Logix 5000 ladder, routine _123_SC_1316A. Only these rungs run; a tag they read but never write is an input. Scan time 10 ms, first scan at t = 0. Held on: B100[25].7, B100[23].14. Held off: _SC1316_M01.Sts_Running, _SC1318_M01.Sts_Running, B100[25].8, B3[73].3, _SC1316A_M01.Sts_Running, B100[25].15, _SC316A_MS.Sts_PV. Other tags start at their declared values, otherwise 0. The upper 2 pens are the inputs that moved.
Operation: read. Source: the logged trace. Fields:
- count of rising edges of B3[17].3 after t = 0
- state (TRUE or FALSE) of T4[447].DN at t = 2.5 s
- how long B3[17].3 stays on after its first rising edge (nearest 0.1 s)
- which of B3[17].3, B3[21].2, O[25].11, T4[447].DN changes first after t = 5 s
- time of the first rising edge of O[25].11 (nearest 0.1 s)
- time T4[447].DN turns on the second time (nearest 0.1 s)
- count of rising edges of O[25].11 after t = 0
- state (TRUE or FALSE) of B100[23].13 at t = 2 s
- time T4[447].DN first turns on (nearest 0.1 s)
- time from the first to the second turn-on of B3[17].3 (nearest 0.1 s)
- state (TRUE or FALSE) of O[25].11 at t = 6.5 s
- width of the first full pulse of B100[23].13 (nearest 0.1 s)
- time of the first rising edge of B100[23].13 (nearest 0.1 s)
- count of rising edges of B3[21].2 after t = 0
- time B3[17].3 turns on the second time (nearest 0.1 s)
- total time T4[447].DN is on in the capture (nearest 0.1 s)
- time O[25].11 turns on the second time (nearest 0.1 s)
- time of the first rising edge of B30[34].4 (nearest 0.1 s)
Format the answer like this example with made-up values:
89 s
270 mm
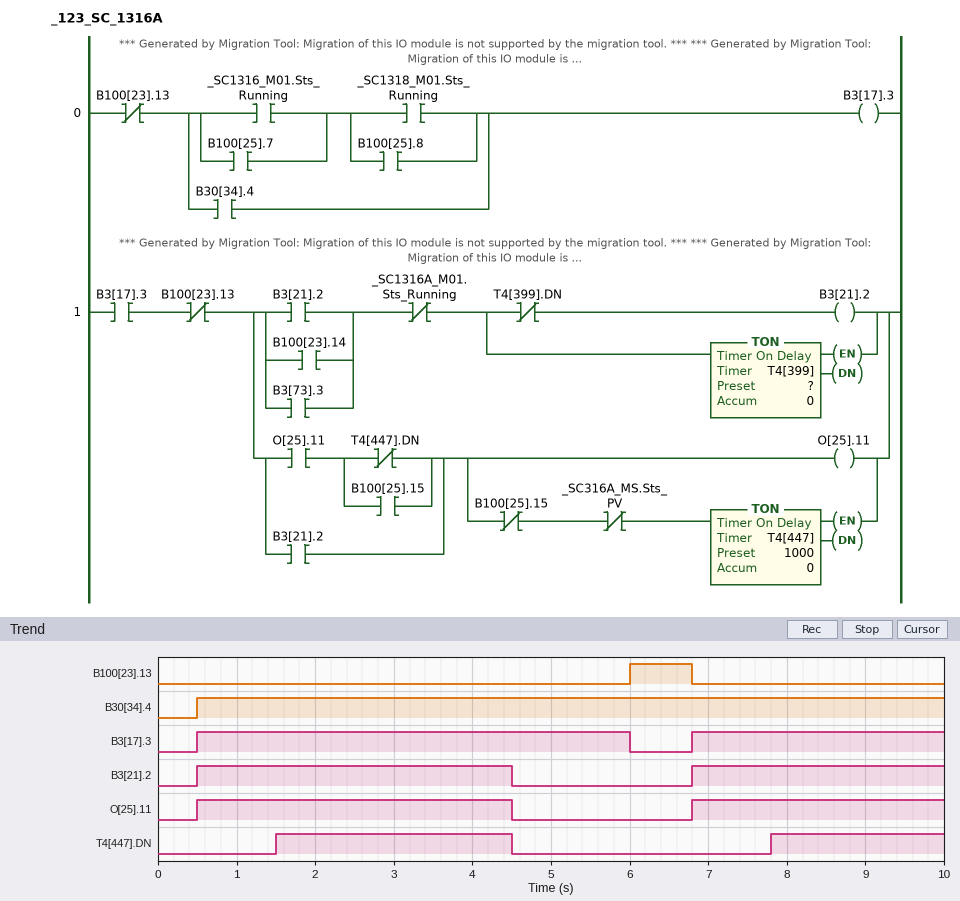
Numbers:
2
TRUE
5.5 s
B3[17].3
0.5 s
7.8 s
2
FALSE
1.5 s
6.3 s
FALSE
0.8 s
6.0 s
2
6.8 s
5.2 s
6.8 s
0.5 s
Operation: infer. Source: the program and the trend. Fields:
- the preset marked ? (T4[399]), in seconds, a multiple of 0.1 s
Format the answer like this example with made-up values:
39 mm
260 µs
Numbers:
4.0 s
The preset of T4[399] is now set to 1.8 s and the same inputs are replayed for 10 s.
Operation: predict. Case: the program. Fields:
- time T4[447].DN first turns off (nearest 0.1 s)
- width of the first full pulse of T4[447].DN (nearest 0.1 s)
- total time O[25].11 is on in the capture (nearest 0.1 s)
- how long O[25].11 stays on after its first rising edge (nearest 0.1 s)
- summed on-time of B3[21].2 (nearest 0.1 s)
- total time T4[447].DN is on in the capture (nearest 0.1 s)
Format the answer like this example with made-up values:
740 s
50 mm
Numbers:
2.3 s
0.8 s
3.6 s
1.8 s
3.6 s
1.6 s
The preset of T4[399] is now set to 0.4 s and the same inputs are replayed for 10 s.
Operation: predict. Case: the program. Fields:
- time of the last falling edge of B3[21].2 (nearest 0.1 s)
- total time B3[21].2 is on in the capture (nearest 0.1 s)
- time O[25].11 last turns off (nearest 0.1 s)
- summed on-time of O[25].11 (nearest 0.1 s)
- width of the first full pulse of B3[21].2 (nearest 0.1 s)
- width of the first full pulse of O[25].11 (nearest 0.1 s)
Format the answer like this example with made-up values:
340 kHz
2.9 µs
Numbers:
7.2 s
0.8 s
7.8 s
2.0 s
0.4 s
1.0 s
